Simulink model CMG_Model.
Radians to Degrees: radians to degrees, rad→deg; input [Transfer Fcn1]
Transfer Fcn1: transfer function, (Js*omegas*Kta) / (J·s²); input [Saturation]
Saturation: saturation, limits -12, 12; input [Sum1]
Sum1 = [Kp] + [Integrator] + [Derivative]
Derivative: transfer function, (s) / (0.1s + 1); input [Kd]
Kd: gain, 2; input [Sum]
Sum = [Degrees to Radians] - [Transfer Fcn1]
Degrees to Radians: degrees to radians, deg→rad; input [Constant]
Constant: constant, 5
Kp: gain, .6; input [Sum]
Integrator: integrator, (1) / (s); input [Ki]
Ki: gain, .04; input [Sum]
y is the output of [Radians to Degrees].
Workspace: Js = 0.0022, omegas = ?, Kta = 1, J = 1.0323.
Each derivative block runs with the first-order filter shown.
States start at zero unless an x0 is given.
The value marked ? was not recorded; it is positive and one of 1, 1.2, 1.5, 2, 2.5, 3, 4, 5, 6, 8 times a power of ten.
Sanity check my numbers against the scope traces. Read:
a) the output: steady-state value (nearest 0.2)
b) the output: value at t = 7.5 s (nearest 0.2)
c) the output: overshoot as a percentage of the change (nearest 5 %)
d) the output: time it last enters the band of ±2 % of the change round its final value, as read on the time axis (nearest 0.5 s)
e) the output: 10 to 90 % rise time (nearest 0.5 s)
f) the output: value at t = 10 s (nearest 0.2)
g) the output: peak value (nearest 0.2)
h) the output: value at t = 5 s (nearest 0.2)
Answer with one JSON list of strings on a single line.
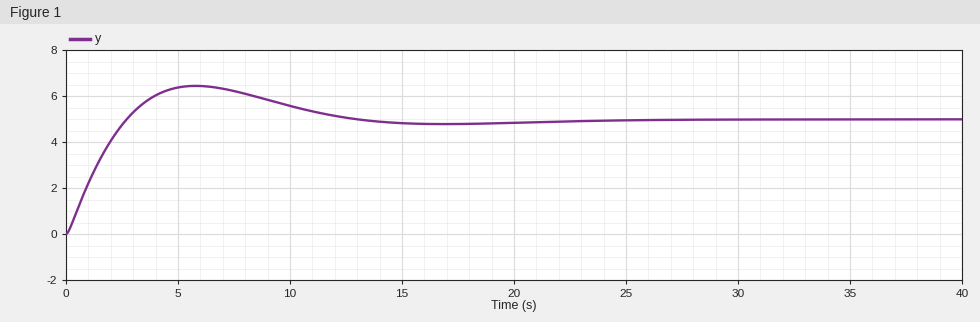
["5.0", "6.2", "30 %", "22.5 s", "2.0 s", "5.6", "6.4", "6.4"]
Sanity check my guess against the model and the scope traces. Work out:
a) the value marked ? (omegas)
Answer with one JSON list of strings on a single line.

["120"]
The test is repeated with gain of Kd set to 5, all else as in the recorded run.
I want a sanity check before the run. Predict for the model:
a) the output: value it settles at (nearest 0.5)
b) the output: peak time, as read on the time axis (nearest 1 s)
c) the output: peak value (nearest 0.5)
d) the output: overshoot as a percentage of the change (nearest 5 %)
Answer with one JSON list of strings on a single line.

["5.0", "4 s", "5.5", "10 %"]
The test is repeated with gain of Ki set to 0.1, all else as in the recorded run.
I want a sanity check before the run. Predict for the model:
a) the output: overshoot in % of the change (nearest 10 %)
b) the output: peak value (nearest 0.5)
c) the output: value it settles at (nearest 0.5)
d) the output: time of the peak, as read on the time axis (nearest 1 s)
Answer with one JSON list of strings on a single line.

["40 %", "7.0", "5.0", "6 s"]
